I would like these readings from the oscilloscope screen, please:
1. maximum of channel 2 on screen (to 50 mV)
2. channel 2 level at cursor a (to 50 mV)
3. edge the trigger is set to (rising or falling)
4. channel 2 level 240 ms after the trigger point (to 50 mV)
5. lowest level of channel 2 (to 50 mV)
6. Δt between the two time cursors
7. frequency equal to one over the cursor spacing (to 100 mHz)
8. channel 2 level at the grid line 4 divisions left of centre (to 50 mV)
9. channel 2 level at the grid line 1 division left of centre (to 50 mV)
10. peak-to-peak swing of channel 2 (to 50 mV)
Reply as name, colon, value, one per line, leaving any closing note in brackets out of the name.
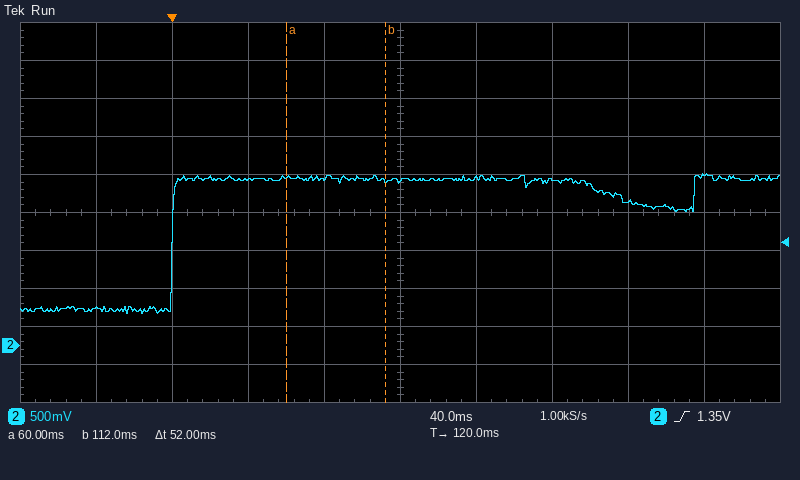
maximum of channel 2 on screen: 2.25 V
channel 2 level at cursor a: 2.20 V
edge the trigger is set to: rising
channel 2 level 240 ms after the trigger point: 1.90 V
lowest level of channel 2: 400 mV
Δt between the two time cursors: 52 ms
frequency equal to one over the cursor spacing: 19.2 Hz
channel 2 level at the grid line 4 divisions left of centre: 500 mV
channel 2 level at the grid line 1 division left of centre: 2.20 V
peak-to-peak swing of channel 2: 1.85 V
